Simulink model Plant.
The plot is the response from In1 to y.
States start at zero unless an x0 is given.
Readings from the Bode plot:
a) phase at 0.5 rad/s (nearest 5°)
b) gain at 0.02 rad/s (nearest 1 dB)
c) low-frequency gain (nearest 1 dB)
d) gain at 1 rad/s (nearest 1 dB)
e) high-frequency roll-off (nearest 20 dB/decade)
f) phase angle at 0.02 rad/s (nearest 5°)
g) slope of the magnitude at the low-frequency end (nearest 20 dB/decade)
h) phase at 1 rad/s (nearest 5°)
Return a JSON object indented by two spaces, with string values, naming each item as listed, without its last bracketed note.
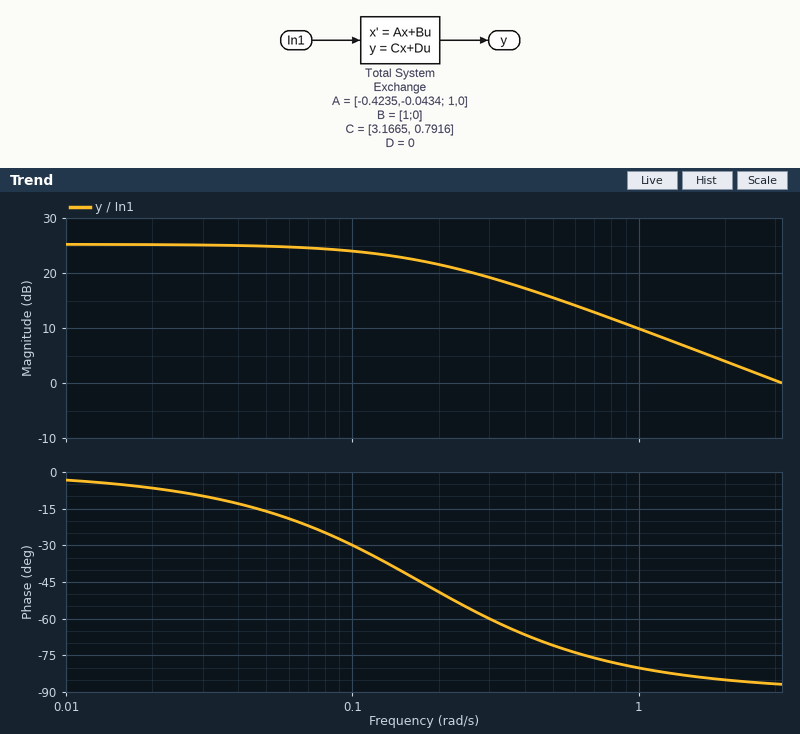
{
  "phase at 0.5 rad/s": "-70°",
  "gain at 0.02 rad/s": "25 dB",
  "low-frequency gain": "25 dB",
  "gain at 1 rad/s": "10 dB",
  "high-frequency roll-off": "-20 dB/decade",
  "phase angle at 0.02 rad/s": "-5°",
  "slope of the magnitude at the low-frequency end": "0 dB/decade",
  "phase at 1 rad/s": "-80°"
}
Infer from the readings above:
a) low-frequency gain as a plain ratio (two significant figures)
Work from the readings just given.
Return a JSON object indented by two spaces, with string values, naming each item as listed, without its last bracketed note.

{
  "low-frequency gain as a plain ratio": "18"
}
